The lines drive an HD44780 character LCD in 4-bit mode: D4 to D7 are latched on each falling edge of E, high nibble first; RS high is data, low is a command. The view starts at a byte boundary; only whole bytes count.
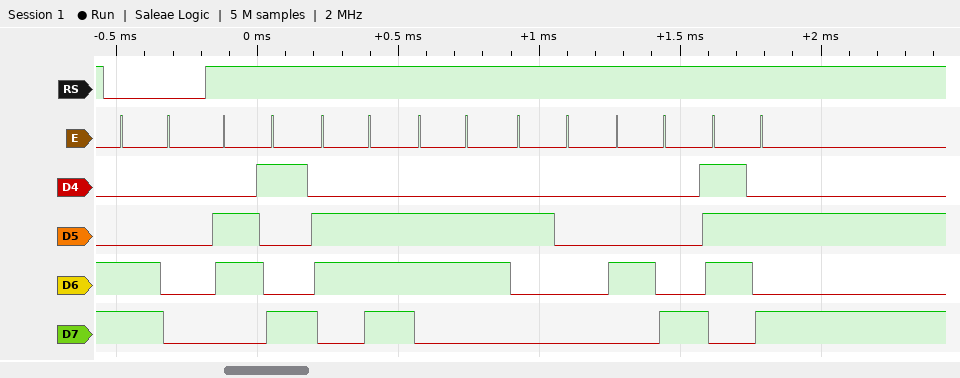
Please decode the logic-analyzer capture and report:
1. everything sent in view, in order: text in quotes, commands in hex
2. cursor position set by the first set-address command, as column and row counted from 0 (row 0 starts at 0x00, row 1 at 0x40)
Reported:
0xC0 "inf Hz"
column 0, row 1
